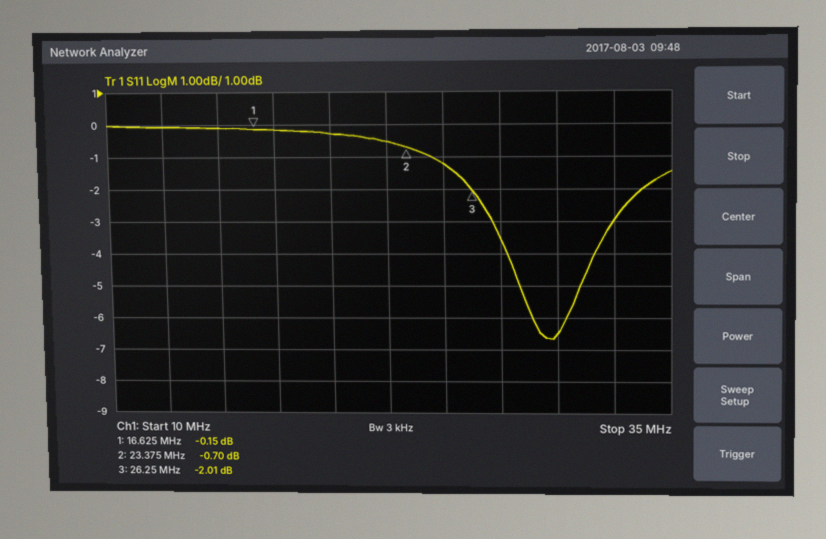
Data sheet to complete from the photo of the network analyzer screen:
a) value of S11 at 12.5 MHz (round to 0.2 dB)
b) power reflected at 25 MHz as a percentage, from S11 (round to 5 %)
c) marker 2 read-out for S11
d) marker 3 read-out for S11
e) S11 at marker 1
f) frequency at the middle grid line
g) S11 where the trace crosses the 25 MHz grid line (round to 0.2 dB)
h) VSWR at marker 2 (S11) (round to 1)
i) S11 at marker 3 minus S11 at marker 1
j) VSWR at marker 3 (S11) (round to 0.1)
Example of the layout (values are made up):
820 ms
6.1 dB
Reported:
0.0 dB
75 %
-0.70 dB
-2.01 dB
-0.15 dB
22.5 MHz
-1.2 dB
25
-1.86 dB
8.7
